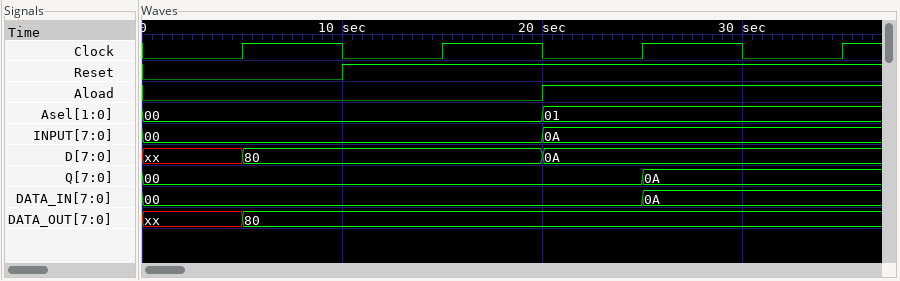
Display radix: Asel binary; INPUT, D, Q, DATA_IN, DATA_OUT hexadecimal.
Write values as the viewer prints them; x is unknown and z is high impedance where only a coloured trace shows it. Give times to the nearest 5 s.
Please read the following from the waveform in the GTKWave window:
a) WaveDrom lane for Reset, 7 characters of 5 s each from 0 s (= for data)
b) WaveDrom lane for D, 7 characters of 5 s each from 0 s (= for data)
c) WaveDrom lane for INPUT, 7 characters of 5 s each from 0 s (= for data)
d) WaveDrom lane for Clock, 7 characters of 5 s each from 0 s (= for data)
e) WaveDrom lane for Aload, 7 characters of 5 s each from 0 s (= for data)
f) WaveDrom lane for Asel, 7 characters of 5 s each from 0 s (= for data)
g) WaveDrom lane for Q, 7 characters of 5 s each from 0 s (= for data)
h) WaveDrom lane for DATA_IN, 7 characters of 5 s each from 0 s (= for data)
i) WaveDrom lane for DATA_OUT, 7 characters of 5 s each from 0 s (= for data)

{name: 'Reset', wave: '0.1....'}
{name: 'D', wave: 'x=..=..', data: '80 0A'}
{name: 'INPUT', wave: '=...=..', data: '00 0A'}
{name: 'Clock', wave: '0101010'}
{name: 'Aload', wave: '0...1..'}
{name: 'Asel', wave: '=...=..', data: '00 01'}
{name: 'Q', wave: '=....=.', data: '00 0A'}
{name: 'DATA_IN', wave: '=....=.', data: '00 0A'}
{name: 'DATA_OUT', wave: 'x=.....', data: '80'}
